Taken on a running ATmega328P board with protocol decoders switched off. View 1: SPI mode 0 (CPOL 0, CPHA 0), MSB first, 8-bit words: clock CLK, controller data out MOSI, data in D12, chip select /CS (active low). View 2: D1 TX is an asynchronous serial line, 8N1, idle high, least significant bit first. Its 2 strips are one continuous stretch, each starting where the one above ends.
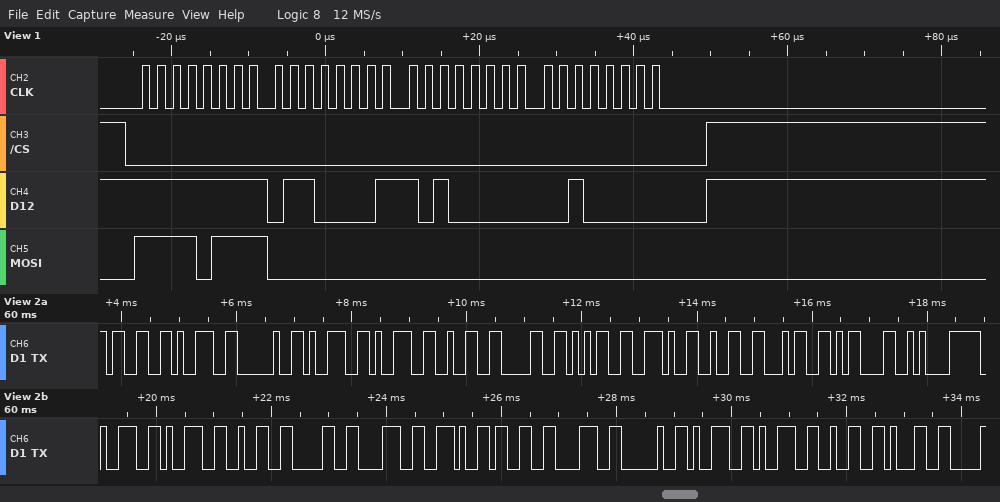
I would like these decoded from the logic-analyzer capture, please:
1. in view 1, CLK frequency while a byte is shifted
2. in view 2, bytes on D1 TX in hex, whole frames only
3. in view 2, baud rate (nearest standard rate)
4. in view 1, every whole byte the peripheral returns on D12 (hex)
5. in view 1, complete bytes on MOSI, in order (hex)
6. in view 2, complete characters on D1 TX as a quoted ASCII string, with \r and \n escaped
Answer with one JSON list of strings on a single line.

["500 kHz", "33 39 20 39 39 32 30 35 2E 32 34 0D 0A 39 39 32 30 38 2E 33 38 20 39 39 32 31", "9600 baud", "0xFF 0x61 0xA0 0x20", "0xF7 0x00 0x00 0x00", "\"39 99205.24\\r\\n99208.38 9921\""]
